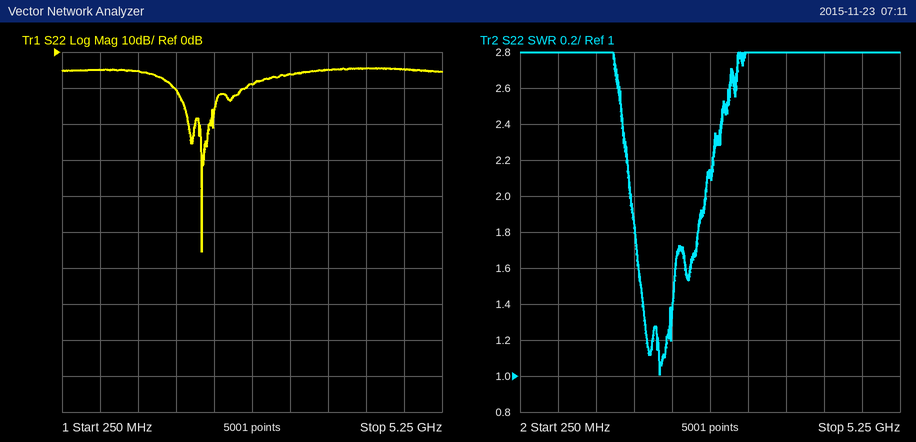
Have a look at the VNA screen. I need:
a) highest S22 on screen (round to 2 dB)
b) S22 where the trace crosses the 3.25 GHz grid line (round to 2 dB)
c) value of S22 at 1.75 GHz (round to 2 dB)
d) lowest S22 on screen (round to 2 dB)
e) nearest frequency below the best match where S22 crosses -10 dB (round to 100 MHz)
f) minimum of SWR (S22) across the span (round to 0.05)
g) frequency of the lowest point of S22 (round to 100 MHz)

-4 dB
-6 dB
-10 dB
-56 dB
1.7 GHz
1.00
2.1 GHz
